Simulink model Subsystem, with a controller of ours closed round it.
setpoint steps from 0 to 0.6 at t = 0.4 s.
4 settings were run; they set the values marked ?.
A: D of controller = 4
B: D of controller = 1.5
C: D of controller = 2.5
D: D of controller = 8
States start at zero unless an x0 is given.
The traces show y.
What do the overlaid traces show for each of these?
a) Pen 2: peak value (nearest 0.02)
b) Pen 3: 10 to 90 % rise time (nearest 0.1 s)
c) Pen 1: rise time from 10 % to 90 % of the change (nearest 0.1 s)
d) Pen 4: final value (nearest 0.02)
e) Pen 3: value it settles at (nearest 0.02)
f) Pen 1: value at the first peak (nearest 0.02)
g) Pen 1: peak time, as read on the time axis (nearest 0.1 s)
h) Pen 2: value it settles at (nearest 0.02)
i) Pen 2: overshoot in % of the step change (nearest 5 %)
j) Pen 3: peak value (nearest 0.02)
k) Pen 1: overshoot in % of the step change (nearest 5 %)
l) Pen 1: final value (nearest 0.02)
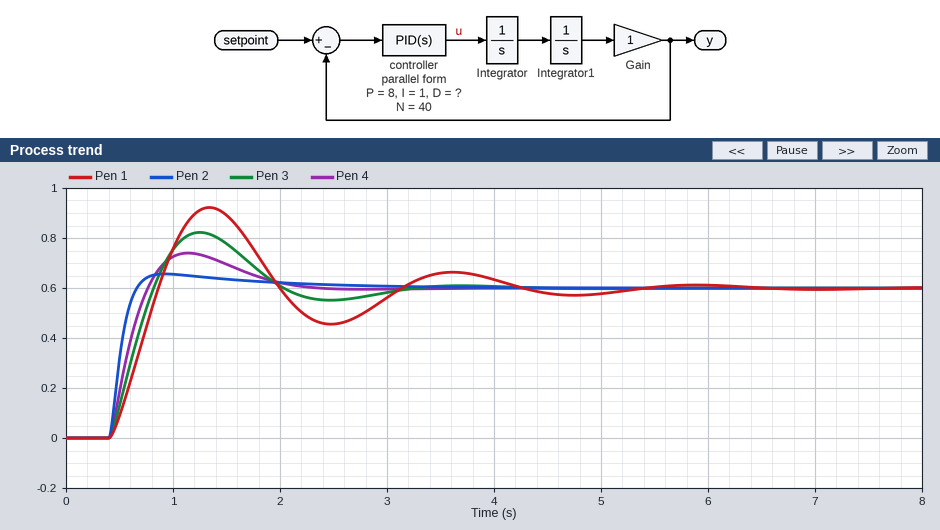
0.66
0.3 s
0.3 s
0.60
0.60
0.92
1.3 s
0.60
10 %
0.82
55 %
0.60
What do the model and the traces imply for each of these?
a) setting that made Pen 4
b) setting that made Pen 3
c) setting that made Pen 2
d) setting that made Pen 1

A
C
D
B
